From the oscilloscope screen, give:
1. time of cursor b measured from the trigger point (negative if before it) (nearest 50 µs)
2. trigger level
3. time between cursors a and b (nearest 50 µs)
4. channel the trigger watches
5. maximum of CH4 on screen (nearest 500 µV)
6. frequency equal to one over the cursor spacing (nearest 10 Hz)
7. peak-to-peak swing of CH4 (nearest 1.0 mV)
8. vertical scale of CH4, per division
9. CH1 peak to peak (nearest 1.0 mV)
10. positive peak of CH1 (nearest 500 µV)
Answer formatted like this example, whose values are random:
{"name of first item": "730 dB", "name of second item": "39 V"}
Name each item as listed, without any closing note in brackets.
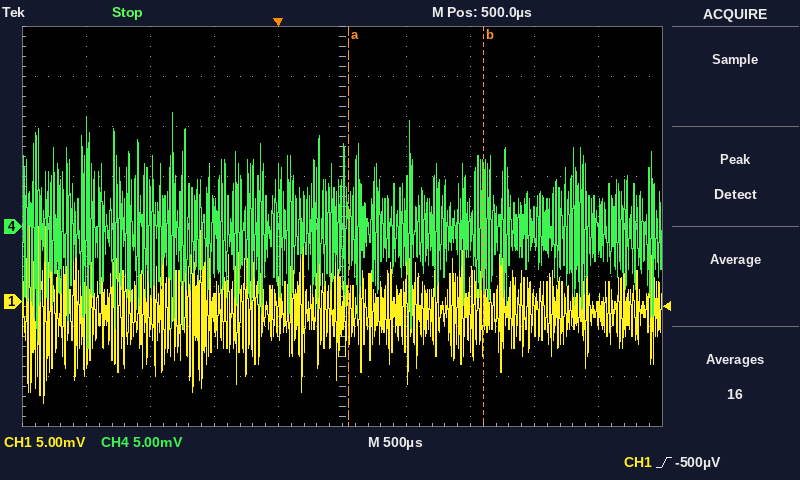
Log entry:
{"time of cursor b measured from the trigger point (negative if before it)": "+1.60 ms", "trigger level": "-500 µV", "time between cursors a and b": "1.05 ms", "channel the trigger watches": "CH1", "maximum of CH4 on screen": "11.5 mV", "frequency equal to one over the cursor spacing": "950 Hz", "peak-to-peak swing of CH4": "24.0 mV", "vertical scale of CH4, per division": "5 mV", "CH1 peak to peak": "18.0 mV", "positive peak of CH1": "7.5 mV"}
